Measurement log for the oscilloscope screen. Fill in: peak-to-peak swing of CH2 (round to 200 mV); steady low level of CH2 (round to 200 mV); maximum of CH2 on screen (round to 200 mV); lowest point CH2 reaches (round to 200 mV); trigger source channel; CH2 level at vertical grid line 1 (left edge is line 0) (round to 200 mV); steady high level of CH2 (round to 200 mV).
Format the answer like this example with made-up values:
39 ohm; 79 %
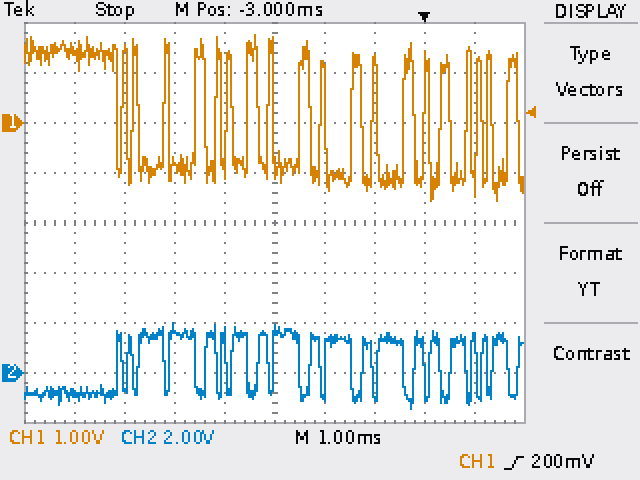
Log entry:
3.4 V; -800 mV; 2.0 V; -1.4 V; CH1; -800 mV; 1.4 V
